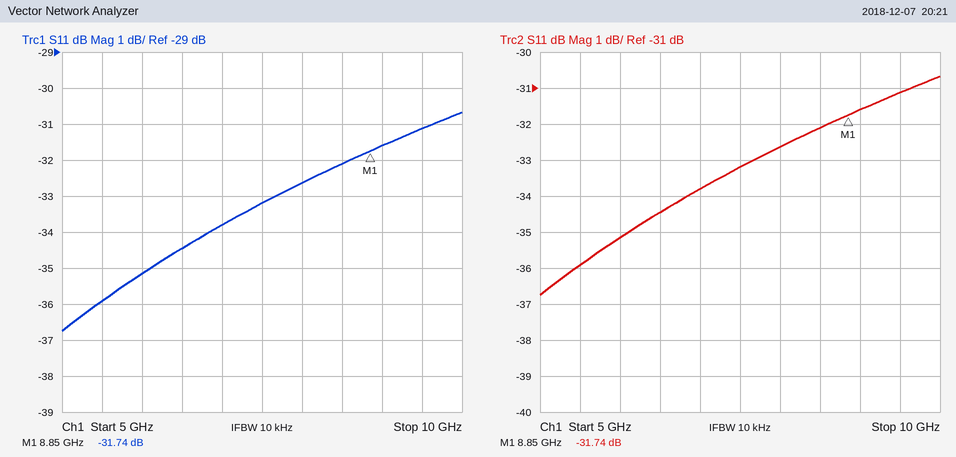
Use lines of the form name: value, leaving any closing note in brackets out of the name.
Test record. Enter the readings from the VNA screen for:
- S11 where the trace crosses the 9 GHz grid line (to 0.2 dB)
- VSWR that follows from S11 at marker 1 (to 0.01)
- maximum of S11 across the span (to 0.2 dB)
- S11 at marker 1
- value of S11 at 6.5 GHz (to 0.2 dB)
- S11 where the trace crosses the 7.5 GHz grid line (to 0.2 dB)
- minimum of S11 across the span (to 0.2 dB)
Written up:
S11 where the trace crosses the 9 GHz grid line: -31.6 dB
VSWR that follows from S11 at marker 1: 1.05
maximum of S11 across the span: -30.6 dB
S11 at marker 1: -31.74 dB
value of S11 at 6.5 GHz: -34.4 dB
S11 where the trace crosses the 7.5 GHz grid line: -33.2 dB
minimum of S11 across the span: -36.8 dB
